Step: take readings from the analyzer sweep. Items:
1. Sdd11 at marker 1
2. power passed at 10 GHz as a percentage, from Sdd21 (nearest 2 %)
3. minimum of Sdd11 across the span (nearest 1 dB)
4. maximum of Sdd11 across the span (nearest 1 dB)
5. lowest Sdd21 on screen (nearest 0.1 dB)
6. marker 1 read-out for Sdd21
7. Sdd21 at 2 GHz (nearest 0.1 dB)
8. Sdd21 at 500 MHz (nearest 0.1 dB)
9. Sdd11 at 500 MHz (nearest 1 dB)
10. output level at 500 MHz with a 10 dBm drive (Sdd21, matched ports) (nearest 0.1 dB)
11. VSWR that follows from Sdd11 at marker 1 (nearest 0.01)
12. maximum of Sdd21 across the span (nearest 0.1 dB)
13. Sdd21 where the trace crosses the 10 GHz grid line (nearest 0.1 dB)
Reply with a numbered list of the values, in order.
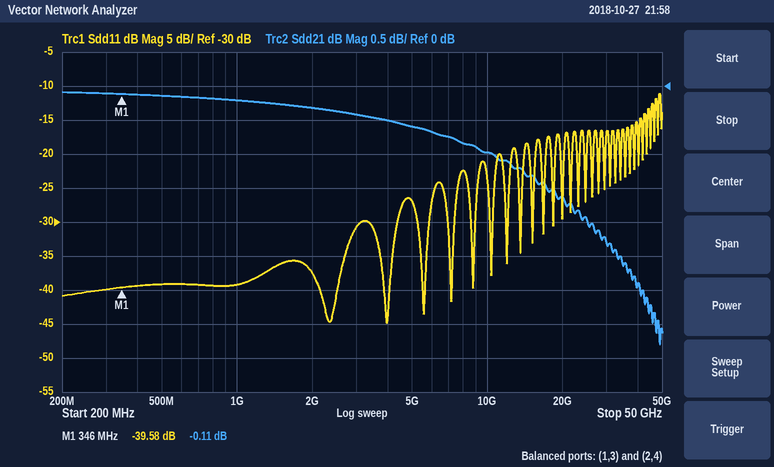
1. -39.58 dB
2. 80 %
3. -45 dB
4. -11 dB
5. -3.8 dB
6. -0.11 dB
7. -0.3 dB
8. -0.1 dB
9. -39 dB
10. 9.9 dBm
11. 1.02
12. -0.1 dB
13. -1.0 dB
